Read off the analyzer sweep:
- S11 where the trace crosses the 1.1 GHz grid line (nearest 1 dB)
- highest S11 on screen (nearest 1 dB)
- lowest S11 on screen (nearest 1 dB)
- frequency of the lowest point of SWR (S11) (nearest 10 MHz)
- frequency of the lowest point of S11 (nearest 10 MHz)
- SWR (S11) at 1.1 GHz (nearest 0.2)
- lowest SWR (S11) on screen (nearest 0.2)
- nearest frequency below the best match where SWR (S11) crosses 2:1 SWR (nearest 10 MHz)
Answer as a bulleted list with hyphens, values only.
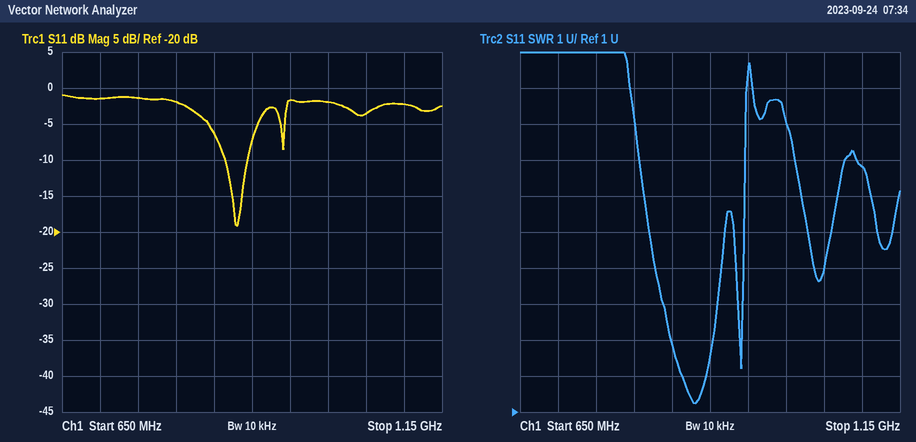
- -2 dB
- -1 dB
- -19 dB
- 880 MHz
- 880 MHz
- 7.8
- 1.2
- 860 MHz
